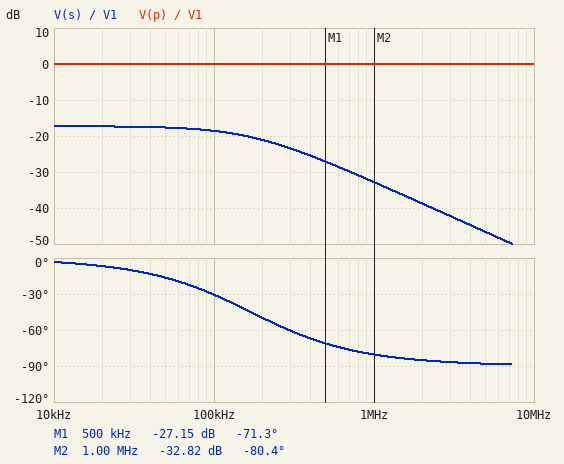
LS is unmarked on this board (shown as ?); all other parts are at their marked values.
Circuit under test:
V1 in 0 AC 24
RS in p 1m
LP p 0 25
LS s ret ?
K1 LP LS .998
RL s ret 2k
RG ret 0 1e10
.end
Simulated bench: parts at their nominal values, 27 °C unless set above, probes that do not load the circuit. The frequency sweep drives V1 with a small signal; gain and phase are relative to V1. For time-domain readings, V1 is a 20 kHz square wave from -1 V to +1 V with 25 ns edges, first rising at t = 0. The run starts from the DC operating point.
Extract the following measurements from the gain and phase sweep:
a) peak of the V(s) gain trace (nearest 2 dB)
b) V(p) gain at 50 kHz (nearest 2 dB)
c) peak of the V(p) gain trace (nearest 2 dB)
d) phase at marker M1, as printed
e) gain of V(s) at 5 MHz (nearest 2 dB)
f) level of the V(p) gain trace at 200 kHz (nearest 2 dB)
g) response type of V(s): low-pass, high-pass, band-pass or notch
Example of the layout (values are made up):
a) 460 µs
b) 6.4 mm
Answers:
a) -18 dB
b) 0 dB
c) 0 dB
d) -71.3 deg
e) -46 dB
f) 0 dB
g) low-pass
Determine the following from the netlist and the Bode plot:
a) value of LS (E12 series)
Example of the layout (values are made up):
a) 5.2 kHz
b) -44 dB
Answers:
a) 470 mH
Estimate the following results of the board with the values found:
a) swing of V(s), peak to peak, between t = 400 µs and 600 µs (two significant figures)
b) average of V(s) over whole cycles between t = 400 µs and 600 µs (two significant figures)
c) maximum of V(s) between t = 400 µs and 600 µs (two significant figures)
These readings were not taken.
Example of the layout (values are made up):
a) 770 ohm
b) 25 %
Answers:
a) 270 mV
b) 140 mV
c) 270 mV
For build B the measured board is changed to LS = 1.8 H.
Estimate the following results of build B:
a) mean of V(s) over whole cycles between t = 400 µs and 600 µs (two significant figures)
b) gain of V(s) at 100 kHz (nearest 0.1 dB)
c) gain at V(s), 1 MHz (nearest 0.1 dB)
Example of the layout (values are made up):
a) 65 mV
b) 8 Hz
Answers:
a) 270 mV
b) -19.3 dB
c) -38.5 dB
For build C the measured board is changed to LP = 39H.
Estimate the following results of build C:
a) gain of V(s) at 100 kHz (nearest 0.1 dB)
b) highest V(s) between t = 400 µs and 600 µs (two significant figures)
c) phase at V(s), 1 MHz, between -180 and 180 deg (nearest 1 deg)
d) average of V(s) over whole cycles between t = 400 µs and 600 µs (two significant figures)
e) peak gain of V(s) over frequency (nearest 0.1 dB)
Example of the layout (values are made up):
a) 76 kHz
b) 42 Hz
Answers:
a) -20.5 dB
b) 220 mV
c) -80 deg
d) 110 mV
e) -19.2 dB
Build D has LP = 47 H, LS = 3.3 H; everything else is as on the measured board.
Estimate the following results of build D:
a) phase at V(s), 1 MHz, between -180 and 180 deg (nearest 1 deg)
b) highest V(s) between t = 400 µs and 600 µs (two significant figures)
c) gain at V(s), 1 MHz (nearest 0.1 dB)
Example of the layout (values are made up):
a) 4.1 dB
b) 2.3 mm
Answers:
a) -89 deg
b) 520 mV
c) -43.9 dB
